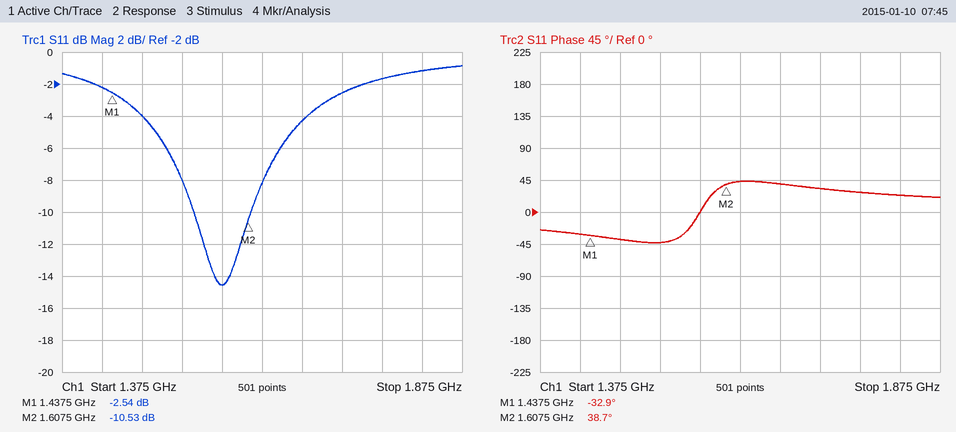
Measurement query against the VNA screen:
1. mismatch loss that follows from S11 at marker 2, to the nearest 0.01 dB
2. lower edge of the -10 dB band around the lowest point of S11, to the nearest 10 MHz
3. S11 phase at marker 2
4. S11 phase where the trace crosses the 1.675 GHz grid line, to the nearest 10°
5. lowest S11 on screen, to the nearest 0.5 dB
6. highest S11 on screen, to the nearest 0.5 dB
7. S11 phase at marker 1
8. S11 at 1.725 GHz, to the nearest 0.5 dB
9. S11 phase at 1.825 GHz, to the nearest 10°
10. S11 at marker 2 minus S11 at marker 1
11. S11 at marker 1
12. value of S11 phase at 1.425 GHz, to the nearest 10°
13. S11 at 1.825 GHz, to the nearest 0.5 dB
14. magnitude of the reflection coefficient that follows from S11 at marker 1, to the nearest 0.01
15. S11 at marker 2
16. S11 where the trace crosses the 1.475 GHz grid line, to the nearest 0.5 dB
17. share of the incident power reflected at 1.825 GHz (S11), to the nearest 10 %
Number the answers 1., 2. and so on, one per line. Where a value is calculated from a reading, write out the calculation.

1. −10 log10(1 − 10^(-10.53/10)) ≈ 0.40 dB
2. 1.54 GHz
3. 38.7°
4. 40°
5. -14.5 dB
6. -1.0 dB
7. -32.9°
8. -2.5 dB
9. 20°
10. -10.53 − (-2.54) = -7.99 dB
11. -2.54 dB
12. -30°
13. -1.0 dB
14. 10^(-2.54/20) ≈ 0.75
15. -10.53 dB
16. -4.0 dB
17. 10^(-1/10) ≈ 79.4 %, so 80 % to the nearest 10 %
